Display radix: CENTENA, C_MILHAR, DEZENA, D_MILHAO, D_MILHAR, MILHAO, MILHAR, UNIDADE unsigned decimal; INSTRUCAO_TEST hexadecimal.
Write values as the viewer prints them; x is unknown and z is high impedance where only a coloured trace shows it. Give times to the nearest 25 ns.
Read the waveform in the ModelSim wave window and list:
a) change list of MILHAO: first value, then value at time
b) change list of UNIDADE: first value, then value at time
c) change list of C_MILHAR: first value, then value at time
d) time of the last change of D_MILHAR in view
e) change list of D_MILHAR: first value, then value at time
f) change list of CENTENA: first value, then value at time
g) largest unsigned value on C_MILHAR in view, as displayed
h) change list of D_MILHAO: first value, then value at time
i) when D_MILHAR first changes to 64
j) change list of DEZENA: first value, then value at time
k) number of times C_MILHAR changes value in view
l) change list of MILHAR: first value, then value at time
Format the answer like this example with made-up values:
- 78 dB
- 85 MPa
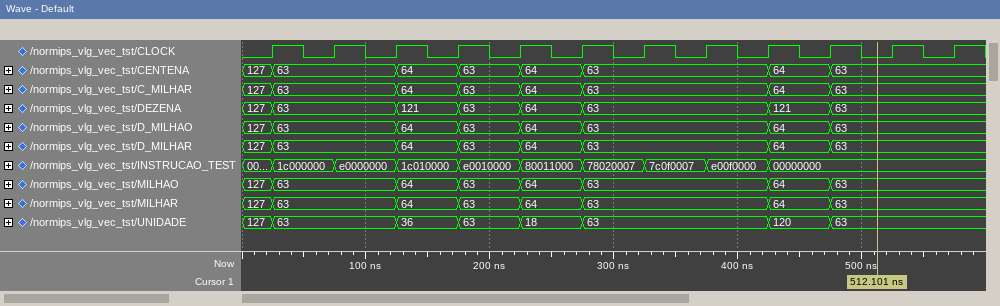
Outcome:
- 127, 63 at 25 ns, 64 at 125 ns, 63 at 175 ns, 64 at 225 ns, 63 at 275 ns, 64 at 425 ns, 63 at 475 ns
- 127, 63 at 25 ns, 36 at 125 ns, 63 at 175 ns, 18 at 225 ns, 63 at 275 ns, 120 at 425 ns, 63 at 475 ns
- 127, 63 at 25 ns, 64 at 125 ns, 63 at 175 ns, 64 at 225 ns, 63 at 275 ns, 64 at 425 ns, 63 at 475 ns
- 475 ns
- 127, 63 at 25 ns, 64 at 125 ns, 63 at 175 ns, 64 at 225 ns, 63 at 275 ns, 64 at 425 ns, 63 at 475 ns
- 127, 63 at 25 ns, 64 at 125 ns, 63 at 175 ns, 64 at 225 ns, 63 at 275 ns, 64 at 425 ns, 63 at 475 ns
- 127
- 127, 63 at 25 ns, 64 at 125 ns, 63 at 175 ns, 64 at 225 ns, 63 at 275 ns, 64 at 425 ns, 63 at 475 ns
- 125 ns
- 127, 63 at 25 ns, 121 at 125 ns, 63 at 175 ns, 64 at 225 ns, 63 at 275 ns, 121 at 425 ns, 63 at 475 ns
- 7
- 127, 63 at 25 ns, 64 at 125 ns, 63 at 175 ns, 64 at 225 ns, 63 at 275 ns, 64 at 425 ns, 63 at 475 ns
